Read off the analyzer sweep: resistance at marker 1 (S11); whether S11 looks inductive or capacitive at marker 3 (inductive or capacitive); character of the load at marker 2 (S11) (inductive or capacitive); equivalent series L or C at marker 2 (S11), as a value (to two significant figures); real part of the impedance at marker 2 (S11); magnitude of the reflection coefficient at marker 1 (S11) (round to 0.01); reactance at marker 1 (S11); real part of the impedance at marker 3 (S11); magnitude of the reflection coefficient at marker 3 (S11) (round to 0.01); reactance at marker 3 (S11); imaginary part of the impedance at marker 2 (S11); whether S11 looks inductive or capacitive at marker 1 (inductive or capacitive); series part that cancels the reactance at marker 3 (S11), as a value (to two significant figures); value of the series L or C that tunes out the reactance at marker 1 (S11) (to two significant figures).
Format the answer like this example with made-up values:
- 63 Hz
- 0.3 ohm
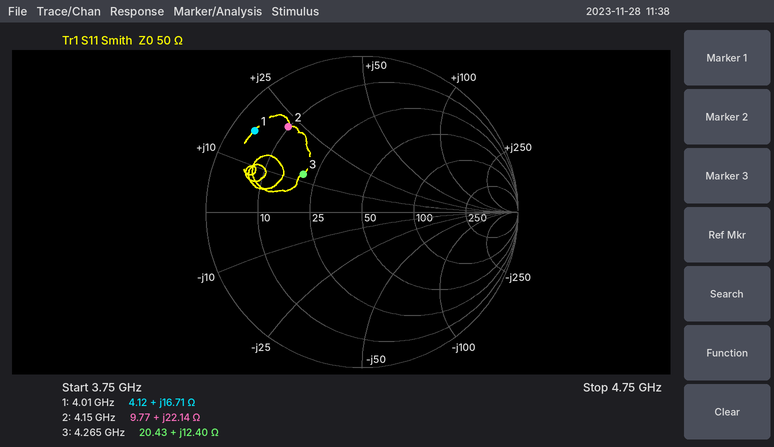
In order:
- 4.12 Ω
- inductive
- inductive
- 850 pH
- 9.77 Ω
- 0.86
- +16.71 Ω
- 20.43 Ω
- 0.45
- +12.40 Ω
- +22.14 Ω
- inductive
- 3.0 pF
- 2.4 pF
